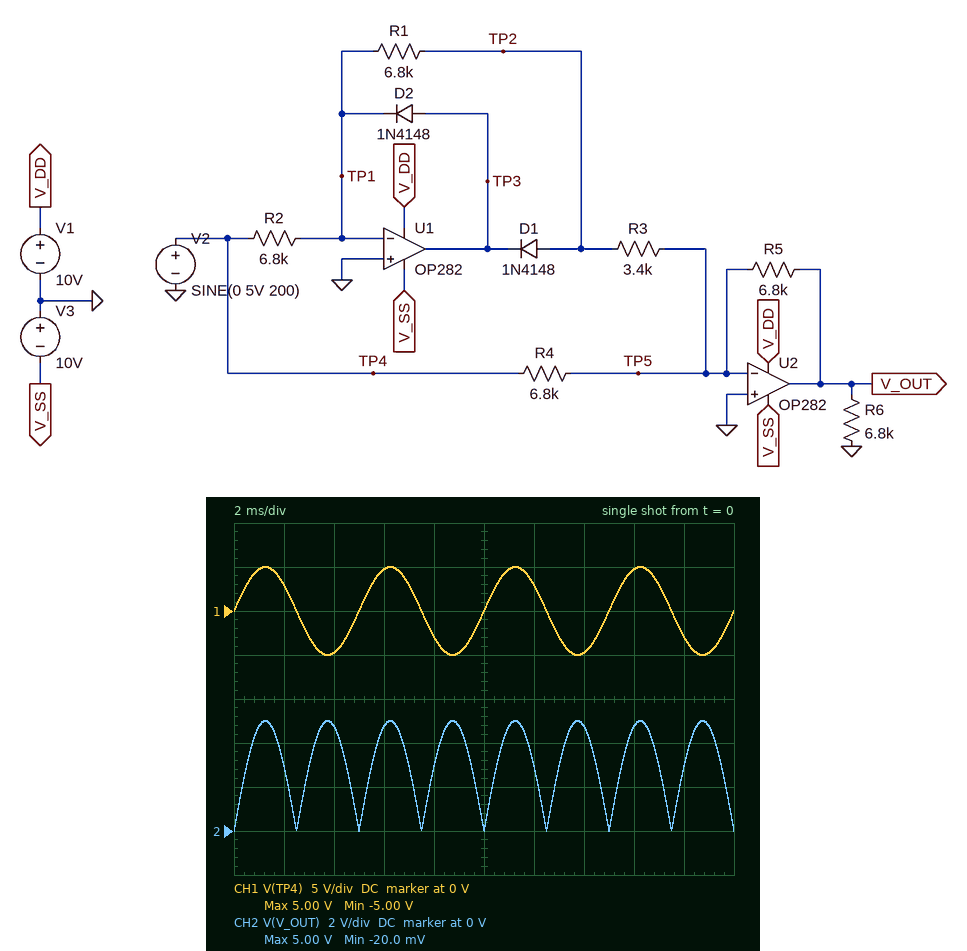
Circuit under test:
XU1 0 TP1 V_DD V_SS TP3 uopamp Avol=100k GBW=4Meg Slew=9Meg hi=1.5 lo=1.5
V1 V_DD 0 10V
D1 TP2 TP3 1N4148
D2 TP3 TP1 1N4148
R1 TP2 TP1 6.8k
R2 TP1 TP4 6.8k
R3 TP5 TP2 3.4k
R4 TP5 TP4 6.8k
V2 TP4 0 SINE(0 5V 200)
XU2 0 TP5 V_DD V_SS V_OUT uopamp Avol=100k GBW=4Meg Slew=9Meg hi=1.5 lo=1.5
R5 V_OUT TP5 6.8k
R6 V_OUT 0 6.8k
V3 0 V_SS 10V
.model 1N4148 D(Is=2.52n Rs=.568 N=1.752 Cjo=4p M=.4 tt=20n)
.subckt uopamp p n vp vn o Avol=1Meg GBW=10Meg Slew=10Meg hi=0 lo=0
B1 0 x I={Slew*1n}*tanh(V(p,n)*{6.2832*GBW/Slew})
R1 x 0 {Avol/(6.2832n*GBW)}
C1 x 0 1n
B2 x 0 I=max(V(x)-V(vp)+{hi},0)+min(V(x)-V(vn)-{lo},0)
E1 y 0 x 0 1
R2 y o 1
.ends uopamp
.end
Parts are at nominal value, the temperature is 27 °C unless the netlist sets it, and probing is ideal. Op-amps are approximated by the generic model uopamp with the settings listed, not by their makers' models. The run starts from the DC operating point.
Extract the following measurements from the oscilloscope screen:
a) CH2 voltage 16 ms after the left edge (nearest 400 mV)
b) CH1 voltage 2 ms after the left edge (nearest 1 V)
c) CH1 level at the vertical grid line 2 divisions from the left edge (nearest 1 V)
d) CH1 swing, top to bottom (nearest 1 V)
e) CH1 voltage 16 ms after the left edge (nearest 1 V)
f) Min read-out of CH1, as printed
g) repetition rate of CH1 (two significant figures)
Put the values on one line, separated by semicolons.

4.8 V; 3 V; -5 V; 10 V; 5 V; -5.00 V; 200 Hz
